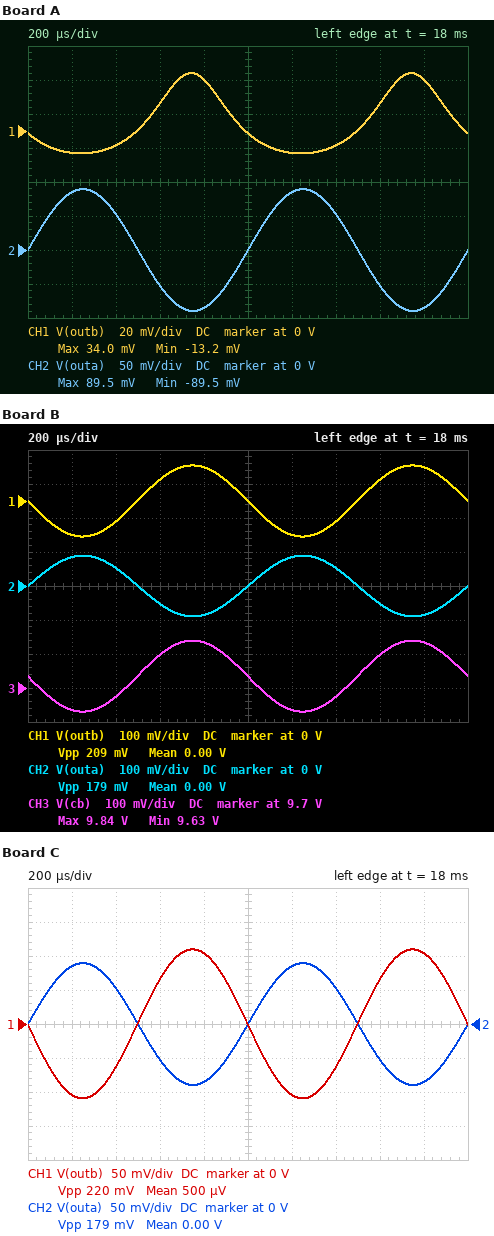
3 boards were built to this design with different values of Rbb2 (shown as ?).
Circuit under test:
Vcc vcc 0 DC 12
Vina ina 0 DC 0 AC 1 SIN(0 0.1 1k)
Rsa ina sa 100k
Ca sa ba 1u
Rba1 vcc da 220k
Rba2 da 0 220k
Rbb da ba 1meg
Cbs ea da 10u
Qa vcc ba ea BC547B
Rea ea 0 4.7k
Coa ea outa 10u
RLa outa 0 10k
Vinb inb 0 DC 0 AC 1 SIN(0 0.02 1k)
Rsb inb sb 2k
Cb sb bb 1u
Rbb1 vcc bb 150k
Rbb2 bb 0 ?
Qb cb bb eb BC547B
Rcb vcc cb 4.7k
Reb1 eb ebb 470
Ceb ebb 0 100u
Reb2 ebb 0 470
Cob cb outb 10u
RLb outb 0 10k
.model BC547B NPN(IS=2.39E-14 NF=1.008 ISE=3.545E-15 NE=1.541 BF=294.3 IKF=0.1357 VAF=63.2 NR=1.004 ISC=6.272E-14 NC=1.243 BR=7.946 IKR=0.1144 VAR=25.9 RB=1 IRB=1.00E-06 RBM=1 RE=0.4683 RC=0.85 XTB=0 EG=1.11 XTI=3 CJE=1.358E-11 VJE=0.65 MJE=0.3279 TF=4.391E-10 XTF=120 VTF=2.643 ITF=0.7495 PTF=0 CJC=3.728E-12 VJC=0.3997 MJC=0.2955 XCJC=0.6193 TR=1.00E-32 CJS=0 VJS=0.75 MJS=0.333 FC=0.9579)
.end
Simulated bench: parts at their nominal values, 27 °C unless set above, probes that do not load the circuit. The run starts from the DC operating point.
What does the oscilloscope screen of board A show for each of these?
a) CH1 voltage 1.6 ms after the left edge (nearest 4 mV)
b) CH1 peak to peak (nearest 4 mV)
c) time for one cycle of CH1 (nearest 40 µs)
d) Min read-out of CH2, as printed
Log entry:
16 mV
48 mV
1.00 ms
-89.5 mV
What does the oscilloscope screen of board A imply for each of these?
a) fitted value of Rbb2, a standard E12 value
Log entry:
56 kΩ
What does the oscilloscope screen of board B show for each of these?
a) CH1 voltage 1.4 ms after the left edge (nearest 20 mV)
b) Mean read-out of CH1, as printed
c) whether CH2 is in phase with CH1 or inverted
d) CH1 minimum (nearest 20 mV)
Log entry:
-60 mV
0.00 V
inverted
-100 mV
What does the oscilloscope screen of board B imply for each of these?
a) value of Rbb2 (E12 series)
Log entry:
15 kΩ
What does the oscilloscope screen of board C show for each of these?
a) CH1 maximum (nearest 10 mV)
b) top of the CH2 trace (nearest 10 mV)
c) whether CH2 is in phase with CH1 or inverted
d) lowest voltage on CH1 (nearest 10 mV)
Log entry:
110 mV
90 mV
inverted
-110 mV
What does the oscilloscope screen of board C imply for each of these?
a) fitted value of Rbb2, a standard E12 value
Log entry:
18 kΩ
